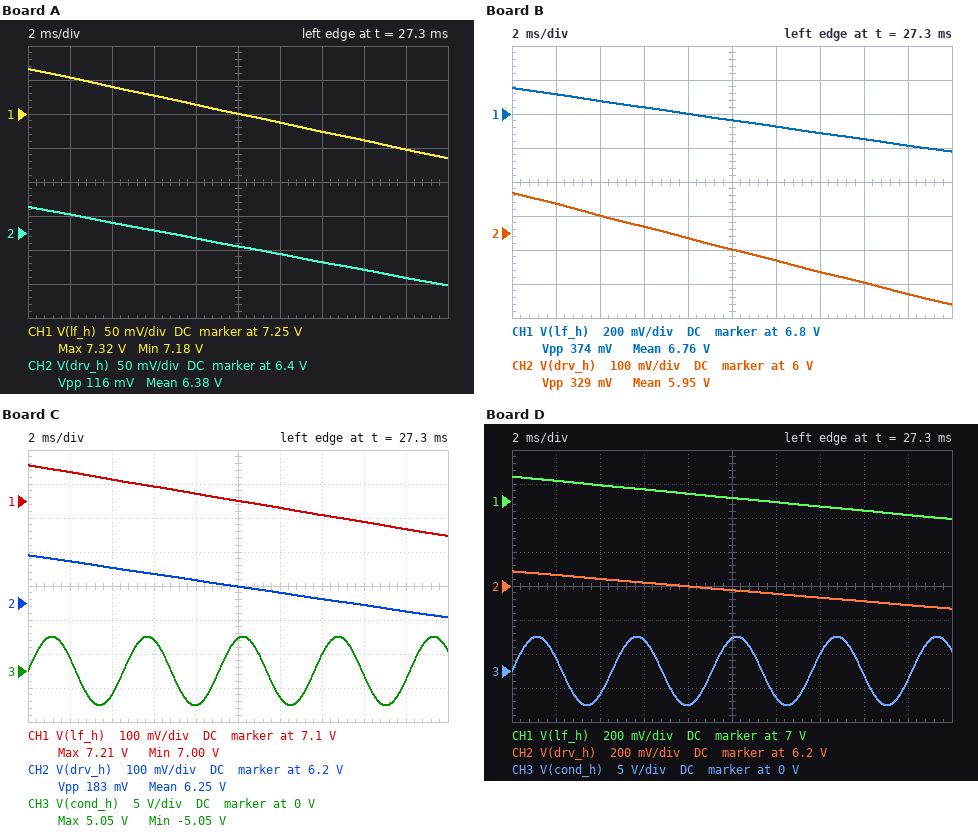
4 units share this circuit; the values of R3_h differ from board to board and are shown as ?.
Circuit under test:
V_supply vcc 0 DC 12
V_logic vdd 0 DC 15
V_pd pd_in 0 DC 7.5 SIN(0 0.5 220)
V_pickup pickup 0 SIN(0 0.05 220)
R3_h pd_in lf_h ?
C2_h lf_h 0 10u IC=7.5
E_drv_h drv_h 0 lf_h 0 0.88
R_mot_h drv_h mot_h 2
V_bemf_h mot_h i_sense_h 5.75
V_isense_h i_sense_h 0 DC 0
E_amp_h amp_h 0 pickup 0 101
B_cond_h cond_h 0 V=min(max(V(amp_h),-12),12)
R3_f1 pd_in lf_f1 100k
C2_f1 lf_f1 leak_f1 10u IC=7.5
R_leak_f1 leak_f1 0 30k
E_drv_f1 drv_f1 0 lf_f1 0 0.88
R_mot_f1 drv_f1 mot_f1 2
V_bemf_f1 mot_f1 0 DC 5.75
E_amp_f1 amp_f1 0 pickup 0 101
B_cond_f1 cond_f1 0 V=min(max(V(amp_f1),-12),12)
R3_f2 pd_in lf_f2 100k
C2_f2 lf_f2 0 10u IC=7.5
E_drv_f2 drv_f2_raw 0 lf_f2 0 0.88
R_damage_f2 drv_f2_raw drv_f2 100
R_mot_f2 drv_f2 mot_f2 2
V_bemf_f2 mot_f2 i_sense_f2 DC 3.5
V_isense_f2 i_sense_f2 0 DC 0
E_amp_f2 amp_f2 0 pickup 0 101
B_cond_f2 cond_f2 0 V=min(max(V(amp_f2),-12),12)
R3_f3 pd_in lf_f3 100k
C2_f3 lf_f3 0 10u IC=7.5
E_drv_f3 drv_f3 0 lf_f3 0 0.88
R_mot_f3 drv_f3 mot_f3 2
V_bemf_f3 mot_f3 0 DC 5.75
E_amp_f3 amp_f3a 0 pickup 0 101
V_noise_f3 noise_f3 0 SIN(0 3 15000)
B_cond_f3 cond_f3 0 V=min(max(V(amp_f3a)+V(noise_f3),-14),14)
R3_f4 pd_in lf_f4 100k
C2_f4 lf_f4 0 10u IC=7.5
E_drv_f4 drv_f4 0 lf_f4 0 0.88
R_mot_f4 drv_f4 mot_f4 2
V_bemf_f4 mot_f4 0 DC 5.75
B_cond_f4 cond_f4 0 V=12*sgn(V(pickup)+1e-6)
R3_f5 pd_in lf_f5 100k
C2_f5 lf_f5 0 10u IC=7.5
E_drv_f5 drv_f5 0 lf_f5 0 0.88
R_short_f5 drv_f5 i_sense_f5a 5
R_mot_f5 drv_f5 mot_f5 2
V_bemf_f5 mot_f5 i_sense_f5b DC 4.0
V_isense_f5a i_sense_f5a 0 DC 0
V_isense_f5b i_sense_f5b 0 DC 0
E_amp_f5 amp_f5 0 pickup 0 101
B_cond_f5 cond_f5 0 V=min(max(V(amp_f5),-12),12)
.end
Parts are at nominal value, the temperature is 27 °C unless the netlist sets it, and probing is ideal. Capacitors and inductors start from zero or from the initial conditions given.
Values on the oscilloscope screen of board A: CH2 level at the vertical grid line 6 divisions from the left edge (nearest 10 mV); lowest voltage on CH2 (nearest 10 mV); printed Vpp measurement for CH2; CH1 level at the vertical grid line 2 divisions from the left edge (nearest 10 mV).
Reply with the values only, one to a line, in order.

6.37 V
6.32 V
116 mV
7.29 V
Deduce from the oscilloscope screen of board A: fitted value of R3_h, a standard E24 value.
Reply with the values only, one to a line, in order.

110 kΩ
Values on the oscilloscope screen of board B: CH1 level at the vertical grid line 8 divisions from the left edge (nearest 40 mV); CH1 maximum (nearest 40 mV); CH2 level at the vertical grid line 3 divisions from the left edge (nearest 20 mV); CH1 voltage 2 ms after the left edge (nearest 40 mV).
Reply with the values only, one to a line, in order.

6.64 V
6.96 V
6.02 V
6.92 V
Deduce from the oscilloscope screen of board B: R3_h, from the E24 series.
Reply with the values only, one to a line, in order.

36 kΩ
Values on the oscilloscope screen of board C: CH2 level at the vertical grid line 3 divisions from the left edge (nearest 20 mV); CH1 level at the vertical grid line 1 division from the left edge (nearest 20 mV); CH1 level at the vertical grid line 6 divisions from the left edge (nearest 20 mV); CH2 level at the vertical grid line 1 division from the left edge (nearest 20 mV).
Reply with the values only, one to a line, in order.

6.28 V
7.18 V
7.08 V
6.32 V
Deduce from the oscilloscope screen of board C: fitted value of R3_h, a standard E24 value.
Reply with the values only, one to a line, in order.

68 kΩ
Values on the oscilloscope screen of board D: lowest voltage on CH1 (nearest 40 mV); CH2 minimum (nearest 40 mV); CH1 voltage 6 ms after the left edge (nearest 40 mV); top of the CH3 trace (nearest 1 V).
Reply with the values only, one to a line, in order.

6.88 V
6.08 V
7.08 V
5 V
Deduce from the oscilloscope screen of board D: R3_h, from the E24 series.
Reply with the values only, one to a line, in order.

56 kΩ
